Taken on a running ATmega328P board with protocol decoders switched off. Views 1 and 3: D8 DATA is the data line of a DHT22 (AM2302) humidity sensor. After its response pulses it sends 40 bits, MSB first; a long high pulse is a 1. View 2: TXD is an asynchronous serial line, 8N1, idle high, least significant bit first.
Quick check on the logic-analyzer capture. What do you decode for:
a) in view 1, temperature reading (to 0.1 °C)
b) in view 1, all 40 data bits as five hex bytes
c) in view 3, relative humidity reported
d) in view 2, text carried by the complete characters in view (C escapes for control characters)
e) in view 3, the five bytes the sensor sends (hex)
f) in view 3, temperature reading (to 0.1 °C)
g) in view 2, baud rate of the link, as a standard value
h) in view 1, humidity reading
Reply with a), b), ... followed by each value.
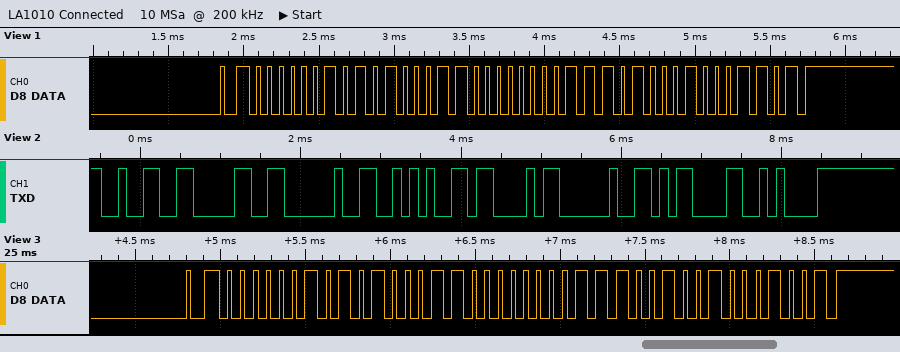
a) 23.2 °C
b) 02 A3 00 E8 8D
c) 67.5 %
d) "20 *C \r\n"
e) 02 A3 00 E4 89
f) 22.8 °C
g) 9600 baud
h) 67.5 %
